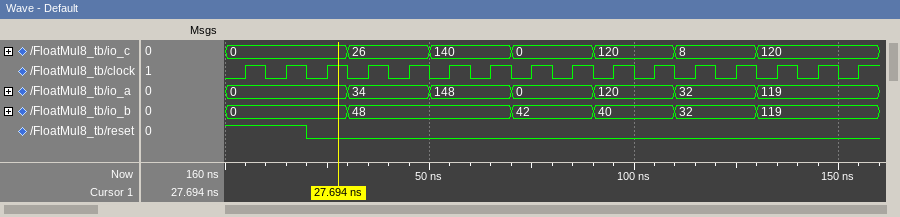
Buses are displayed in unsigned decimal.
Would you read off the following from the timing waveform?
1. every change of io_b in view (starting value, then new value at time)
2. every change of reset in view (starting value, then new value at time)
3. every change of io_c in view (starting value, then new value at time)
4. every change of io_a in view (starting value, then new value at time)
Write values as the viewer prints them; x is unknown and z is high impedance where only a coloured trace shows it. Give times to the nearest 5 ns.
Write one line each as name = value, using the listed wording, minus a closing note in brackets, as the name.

every change of io_b in view = 0, 48 at 30 ns, 42 at 70 ns, 40 at 90 ns, 32 at 110 ns, 119 at 130 ns
every change of reset in view = 1, 0 at 20 ns
every change of io_c in view = 0, 26 at 30 ns, 140 at 50 ns, 0 at 70 ns, 120 at 90 ns, 8 at 110 ns, 120 at 130 ns
every change of io_a in view = 0, 34 at 30 ns, 148 at 50 ns, 0 at 70 ns, 120 at 90 ns, 32 at 110 ns, 119 at 130 ns
